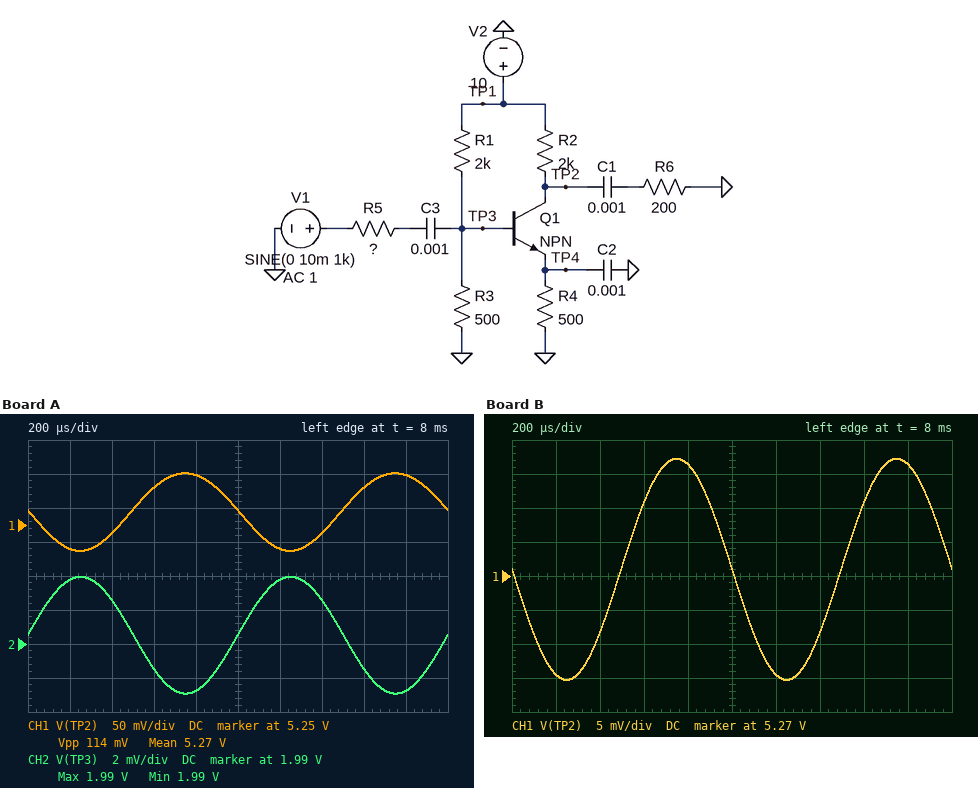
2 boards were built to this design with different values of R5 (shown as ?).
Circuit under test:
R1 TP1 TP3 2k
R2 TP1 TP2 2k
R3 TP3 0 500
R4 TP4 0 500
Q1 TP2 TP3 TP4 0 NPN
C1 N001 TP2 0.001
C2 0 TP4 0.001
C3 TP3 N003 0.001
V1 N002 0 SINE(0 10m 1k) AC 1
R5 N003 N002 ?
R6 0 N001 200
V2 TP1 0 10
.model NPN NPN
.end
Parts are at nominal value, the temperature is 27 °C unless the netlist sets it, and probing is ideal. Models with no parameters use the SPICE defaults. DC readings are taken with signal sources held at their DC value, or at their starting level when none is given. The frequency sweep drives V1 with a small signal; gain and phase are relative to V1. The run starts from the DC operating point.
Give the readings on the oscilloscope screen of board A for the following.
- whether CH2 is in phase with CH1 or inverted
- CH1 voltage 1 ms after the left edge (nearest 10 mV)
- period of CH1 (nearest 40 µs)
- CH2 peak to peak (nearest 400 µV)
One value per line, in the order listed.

inverted
5.27 V
1.00 ms
6.8 mV
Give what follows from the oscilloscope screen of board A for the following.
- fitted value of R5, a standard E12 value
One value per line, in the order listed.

560 Ω
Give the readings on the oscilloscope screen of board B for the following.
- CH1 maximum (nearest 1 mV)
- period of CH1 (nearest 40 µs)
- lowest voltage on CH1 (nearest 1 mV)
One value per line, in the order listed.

5.287 V
1.00 ms
5.255 V
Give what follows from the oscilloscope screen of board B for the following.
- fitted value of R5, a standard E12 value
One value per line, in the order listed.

2.7 kΩ
